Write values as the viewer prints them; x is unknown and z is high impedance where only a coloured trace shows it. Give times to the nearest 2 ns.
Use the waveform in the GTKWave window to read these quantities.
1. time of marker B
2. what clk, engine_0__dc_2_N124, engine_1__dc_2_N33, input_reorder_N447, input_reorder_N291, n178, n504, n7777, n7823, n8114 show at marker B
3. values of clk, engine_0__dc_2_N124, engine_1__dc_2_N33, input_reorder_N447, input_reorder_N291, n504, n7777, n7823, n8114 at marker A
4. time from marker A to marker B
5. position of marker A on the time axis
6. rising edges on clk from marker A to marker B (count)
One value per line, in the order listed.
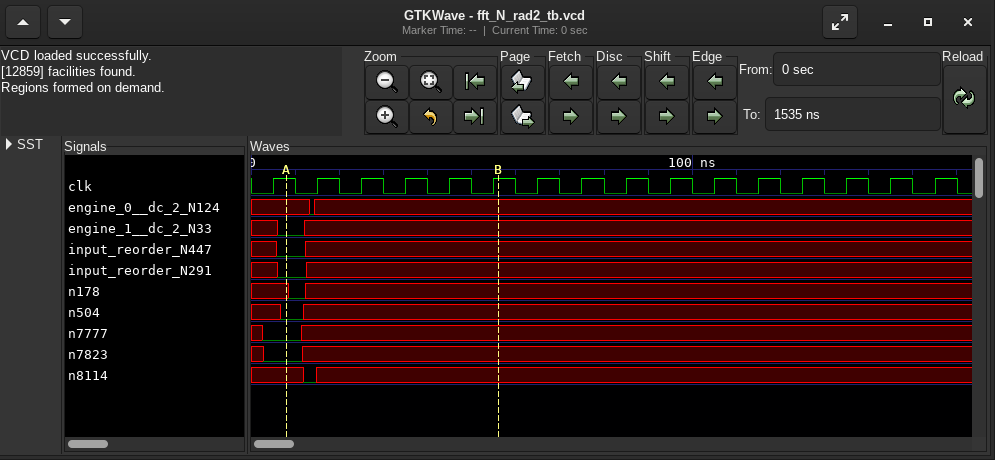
56 ns
clk=1, engine_0__dc_2_N124=x, engine_1__dc_2_N33=x, input_reorder_N447=x, input_reorder_N291=x, n178=x, n504=x, n7777=x, n7823=x, n8114=x
clk=1, engine_0__dc_2_N124=x, engine_1__dc_2_N33=0, input_reorder_N447=0, input_reorder_N291=0, n504=0, n7777=0, n7823=0, n8114=x
48 ns
8 ns
5
